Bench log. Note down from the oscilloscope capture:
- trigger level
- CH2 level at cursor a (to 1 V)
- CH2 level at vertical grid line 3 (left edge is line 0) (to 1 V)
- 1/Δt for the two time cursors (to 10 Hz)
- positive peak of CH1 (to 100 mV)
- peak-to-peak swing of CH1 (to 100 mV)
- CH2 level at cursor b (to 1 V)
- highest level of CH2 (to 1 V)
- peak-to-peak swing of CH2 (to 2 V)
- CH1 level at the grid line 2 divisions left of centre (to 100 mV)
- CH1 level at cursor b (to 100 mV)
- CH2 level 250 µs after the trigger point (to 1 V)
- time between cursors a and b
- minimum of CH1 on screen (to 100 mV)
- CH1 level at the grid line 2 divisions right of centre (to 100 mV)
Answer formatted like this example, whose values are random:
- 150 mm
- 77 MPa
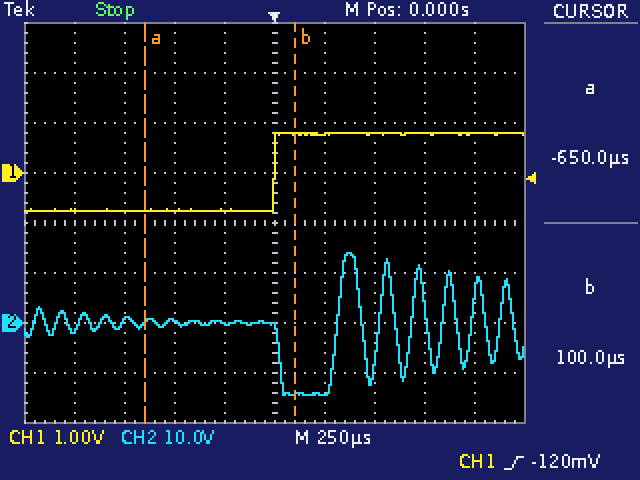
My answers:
- -120 mV
- 0 V
- 0 V
- 1.33 kHz
- 800 mV
- 1.6 V
- -14 V
- 14 V
- 28 V
- -800 mV
- 800 mV
- -14 V
- 750 µs
- -800 mV
- 800 mV
